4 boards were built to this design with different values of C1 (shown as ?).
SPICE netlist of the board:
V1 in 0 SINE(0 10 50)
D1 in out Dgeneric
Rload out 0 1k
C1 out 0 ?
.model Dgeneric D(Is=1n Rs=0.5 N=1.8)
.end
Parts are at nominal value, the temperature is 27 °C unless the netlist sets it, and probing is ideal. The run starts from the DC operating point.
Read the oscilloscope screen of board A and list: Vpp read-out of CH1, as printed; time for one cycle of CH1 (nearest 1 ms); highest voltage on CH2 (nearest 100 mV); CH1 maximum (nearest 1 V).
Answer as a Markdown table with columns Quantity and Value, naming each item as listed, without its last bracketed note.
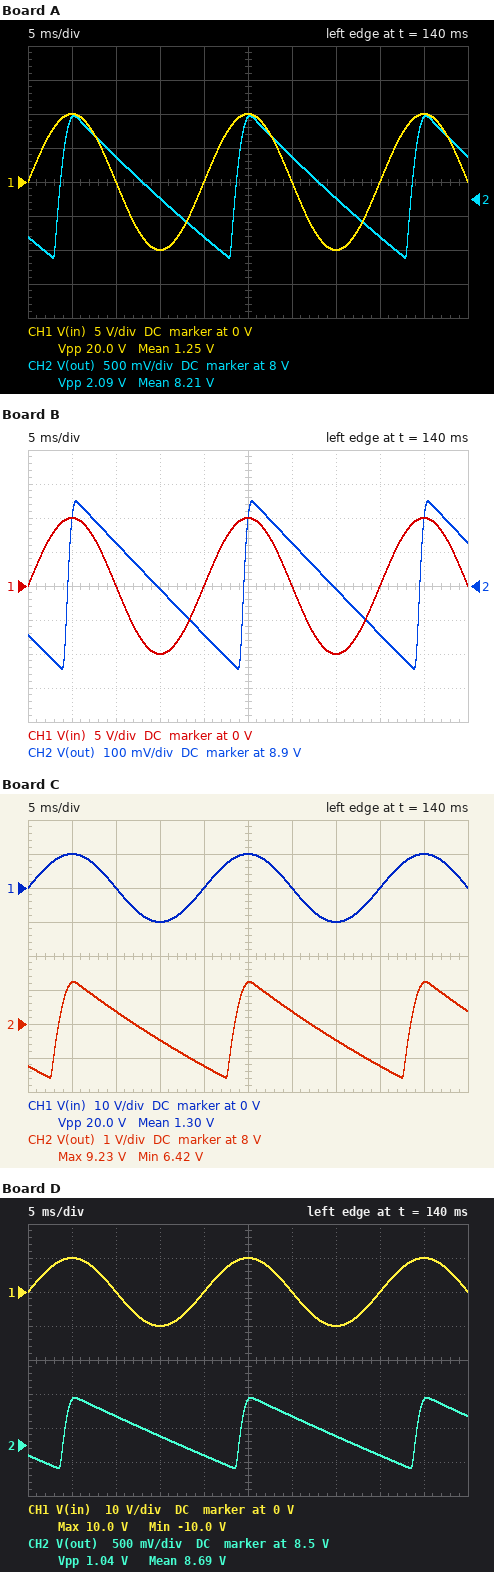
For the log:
| Quantity | Value |
|---|---|
| Vpp read-out of CH1, as printed | 20.0 V |
| time for one cycle of CH1 | 20 ms |
| highest voltage on CH2 | 9.2 V |
| CH1 maximum | 10 V |
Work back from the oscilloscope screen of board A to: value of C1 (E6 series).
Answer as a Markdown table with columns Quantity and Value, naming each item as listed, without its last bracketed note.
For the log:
| Quantity | Value |
|---|---|
| value of C1 | 68 µF |
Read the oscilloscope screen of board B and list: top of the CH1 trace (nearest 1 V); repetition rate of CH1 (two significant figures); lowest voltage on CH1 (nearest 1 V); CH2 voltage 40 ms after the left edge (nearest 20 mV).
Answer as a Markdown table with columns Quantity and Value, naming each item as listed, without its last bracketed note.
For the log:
| Quantity | Value |
|---|---|
| top of the CH1 trace | 10 V |
| repetition rate of CH1 | 50 Hz |
| lowest voltage on CH1 | -10 V |
| CH2 voltage 40 ms after the left edge | 8.76 V |
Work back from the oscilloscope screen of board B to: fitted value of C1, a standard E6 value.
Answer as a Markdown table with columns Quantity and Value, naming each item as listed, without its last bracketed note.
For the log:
| Quantity | Value |
|---|---|
| fitted value of C1, a standard E6 value | 330 µF |
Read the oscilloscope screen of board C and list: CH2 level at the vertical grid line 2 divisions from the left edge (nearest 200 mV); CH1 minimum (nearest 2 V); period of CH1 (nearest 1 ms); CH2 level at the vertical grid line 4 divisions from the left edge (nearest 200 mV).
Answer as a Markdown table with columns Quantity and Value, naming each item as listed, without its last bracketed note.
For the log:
| Quantity | Value |
|---|---|
| CH2 level at the vertical grid line 2 divisions from the left edge | 8.4 V |
| CH1 minimum | -10 V |
| period of CH1 | 20 ms |
| CH2 level at the vertical grid line 4 divisions from the left edge | 6.8 V |
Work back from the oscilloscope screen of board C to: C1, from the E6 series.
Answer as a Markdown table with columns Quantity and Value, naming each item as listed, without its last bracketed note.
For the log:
| Quantity | Value |
|---|---|
| C1, from the E6 series | 47 µF |
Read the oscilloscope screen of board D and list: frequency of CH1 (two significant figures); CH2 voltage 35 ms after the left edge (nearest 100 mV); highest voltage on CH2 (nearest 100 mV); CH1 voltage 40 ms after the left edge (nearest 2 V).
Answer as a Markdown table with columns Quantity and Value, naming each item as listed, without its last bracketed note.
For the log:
| Quantity | Value |
|---|---|
| frequency of CH1 | 50 Hz |
| CH2 voltage 35 ms after the left edge | 8.6 V |
| highest voltage on CH2 | 9.2 V |
| CH1 voltage 40 ms after the left edge | 0 V |
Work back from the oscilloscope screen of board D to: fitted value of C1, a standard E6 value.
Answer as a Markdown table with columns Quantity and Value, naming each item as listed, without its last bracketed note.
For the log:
| Quantity | Value |
|---|---|
| fitted value of C1, a standard E6 value | 150 µF |
